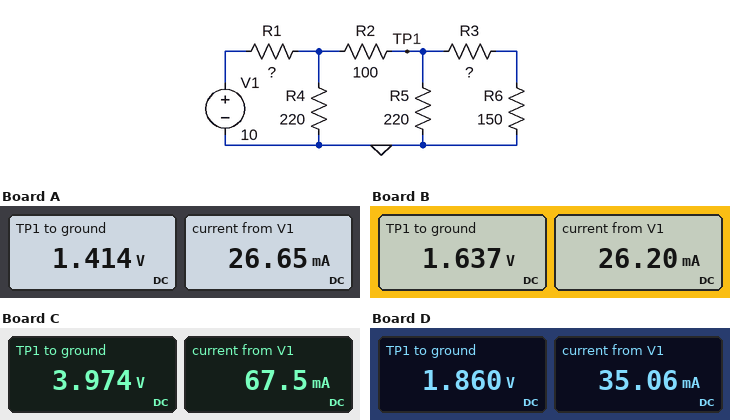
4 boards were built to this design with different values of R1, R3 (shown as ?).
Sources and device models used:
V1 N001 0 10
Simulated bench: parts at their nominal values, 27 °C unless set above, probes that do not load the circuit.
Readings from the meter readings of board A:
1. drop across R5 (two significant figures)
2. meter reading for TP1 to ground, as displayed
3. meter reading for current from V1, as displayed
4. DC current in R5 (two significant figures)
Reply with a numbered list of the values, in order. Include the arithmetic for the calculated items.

1. 1.414 V = 1.4 V
2. 1.414 V
3. 26.65 mA
4. (1.414 V) / 220 Ω = 6.4 mA
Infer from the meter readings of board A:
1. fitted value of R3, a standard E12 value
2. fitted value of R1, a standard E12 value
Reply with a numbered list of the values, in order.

1. 39 Ω
2. 270 Ω
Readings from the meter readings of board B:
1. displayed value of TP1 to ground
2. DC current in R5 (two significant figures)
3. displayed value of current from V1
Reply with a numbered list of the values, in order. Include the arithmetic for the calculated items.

1. 1.637 V
2. (1.637 V) / 220 Ω = 7.4 mA
3. 26.20 mA
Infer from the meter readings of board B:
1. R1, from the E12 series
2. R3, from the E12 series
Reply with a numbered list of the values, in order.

1. 270 Ω
2. 150 Ω
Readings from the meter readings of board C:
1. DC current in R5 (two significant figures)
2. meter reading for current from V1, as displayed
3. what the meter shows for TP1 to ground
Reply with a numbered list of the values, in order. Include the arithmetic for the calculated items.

1. (3.974 V) / 220 Ω = 18 mA
2. 67.5 mA
3. 3.974 V
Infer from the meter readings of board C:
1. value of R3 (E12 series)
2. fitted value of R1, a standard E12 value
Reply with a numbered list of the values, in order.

1. 100 Ω
2. 39 Ω
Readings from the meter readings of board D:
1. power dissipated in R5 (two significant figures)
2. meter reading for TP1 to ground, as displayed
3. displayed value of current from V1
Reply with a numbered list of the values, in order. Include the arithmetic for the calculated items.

1. (1.86 V)^2 / 220 Ω = 16 mW
2. 1.860 V
3. 35.06 mA
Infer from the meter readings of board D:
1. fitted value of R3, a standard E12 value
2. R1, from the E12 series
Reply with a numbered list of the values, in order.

1. 39 Ω
2. 180 Ω
